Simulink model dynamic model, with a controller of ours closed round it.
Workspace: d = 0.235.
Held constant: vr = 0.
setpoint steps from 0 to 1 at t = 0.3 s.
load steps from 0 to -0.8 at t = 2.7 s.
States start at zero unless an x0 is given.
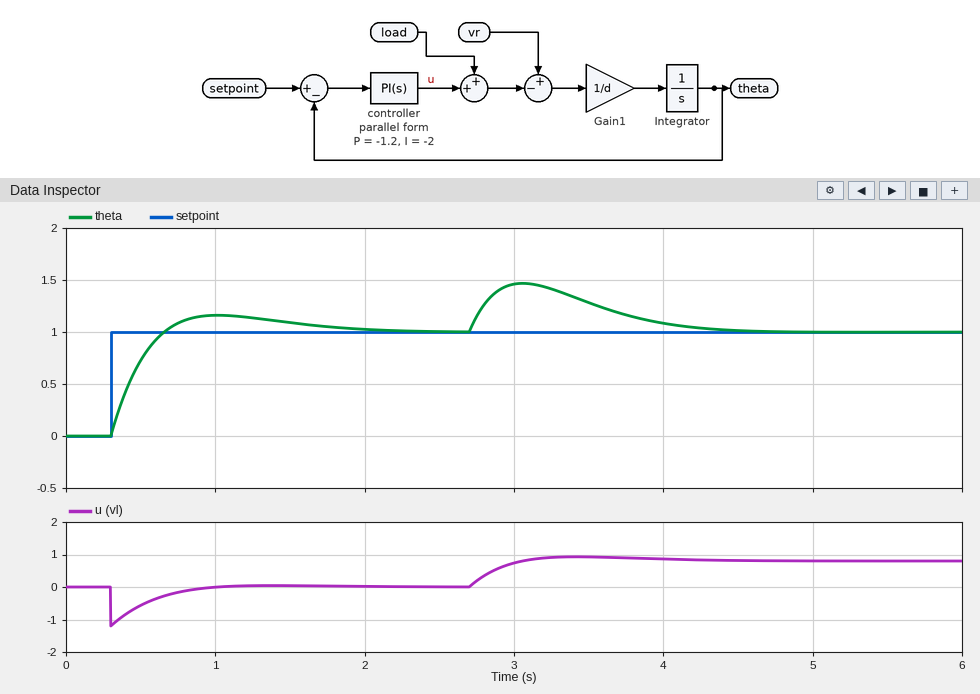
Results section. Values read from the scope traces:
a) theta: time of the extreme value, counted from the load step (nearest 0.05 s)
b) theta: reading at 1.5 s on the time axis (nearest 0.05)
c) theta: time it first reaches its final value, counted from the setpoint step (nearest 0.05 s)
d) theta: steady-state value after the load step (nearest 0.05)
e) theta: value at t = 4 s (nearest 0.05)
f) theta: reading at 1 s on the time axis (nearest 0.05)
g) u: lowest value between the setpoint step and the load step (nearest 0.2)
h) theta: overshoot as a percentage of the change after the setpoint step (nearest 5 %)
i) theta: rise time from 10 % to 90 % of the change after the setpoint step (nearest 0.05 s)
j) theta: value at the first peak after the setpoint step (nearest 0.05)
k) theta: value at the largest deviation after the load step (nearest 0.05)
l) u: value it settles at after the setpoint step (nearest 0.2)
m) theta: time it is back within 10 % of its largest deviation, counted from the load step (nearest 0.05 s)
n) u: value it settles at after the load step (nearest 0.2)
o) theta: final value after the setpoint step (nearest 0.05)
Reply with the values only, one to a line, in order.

0.35 s
1.10
0.35 s
1.00
1.10
1.15
-1.2
15 %
0.25 s
1.15
1.45
0.0
1.50 s
0.8
1.00
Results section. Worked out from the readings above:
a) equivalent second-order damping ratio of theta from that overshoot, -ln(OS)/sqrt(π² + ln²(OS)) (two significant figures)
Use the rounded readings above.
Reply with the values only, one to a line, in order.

0.52
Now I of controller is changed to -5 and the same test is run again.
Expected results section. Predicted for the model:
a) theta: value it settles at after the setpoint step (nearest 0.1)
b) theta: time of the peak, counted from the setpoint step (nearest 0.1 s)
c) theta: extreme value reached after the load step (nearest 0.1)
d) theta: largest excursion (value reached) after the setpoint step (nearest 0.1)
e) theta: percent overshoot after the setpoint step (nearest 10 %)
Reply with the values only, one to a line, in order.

1.0
0.5 s
1.4
1.3
30 %
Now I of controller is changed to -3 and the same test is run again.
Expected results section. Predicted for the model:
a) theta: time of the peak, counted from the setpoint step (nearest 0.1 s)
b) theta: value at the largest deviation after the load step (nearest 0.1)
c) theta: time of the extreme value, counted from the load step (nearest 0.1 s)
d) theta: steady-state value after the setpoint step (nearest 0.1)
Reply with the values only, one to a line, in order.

0.6 s
1.4
0.3 s
1.0
